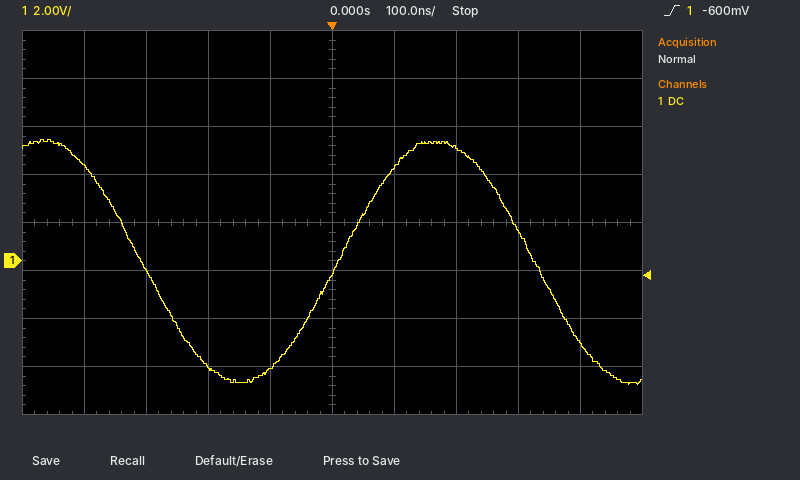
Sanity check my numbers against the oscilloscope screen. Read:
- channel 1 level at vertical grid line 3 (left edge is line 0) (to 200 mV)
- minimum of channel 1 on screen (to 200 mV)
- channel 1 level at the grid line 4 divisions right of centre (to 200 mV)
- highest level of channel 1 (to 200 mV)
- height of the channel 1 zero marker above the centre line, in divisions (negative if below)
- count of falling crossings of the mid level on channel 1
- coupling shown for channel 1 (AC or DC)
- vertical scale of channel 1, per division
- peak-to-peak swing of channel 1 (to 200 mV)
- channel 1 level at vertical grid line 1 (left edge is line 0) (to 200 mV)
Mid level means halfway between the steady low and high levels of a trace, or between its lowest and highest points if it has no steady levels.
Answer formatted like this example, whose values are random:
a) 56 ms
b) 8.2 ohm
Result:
a) -4.4 V
b) -5.2 V
c) -3.4 V
d) 5.0 V
e) -0.8 div
f) 2
g) DC
h) 2 V
i) 10.2 V
j) 4.0 V
